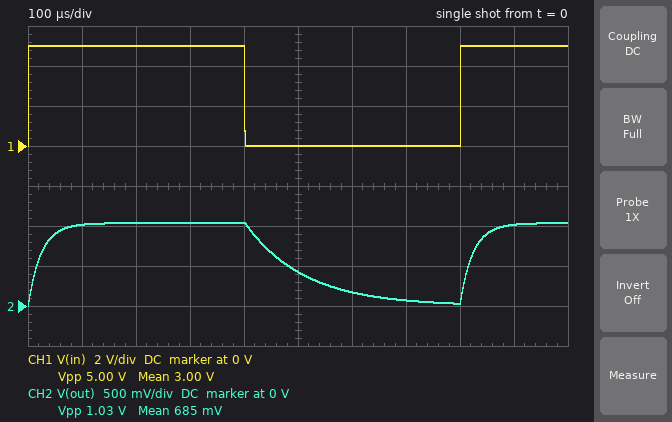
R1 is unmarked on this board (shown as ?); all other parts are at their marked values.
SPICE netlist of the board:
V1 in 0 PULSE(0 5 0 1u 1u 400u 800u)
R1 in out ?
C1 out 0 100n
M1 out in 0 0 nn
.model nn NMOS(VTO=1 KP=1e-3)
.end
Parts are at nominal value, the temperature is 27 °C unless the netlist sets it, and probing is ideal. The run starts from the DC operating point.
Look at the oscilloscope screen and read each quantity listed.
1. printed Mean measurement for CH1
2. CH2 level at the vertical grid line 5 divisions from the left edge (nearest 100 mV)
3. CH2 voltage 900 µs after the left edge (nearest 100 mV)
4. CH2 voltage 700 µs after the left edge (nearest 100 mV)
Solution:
3.00 V
400 mV
1.0 V
100 mV
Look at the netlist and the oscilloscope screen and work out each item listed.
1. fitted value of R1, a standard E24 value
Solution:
1.1 kΩ
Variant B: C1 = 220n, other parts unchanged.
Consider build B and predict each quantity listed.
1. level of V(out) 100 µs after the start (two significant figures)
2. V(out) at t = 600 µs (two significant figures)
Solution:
870 mV
460 mV
